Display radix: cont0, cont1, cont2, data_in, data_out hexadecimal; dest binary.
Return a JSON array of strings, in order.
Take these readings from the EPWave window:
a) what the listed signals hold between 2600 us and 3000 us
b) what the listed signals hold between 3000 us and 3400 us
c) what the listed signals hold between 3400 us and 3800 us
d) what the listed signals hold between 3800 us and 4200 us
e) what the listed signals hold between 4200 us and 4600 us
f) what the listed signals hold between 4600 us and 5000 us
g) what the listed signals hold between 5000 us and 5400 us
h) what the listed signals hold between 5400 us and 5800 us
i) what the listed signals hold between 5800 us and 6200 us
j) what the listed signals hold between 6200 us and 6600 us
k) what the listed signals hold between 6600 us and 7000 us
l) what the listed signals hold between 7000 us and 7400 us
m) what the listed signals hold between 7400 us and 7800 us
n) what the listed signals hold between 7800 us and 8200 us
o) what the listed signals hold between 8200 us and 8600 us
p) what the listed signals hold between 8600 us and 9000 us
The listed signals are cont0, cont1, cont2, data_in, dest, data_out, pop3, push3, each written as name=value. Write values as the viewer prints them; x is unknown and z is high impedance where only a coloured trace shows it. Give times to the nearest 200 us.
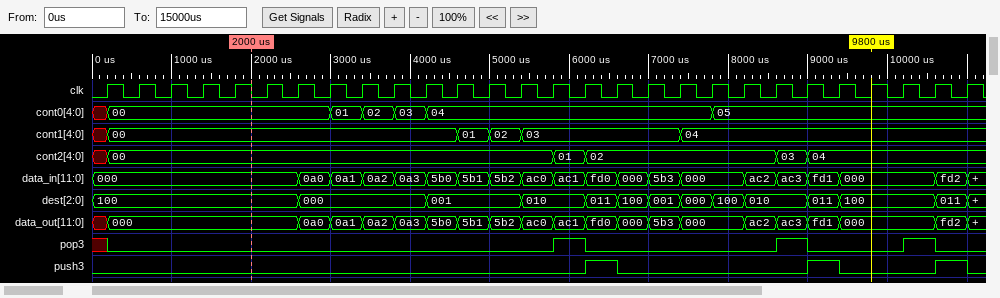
["cont0=00, cont1=00, cont2=00, data_in=0a0, dest=000, data_out=0a0, pop3=0, push3=0", "cont0=01, cont1=00, cont2=00, data_in=0a1, dest=000, data_out=0a1, pop3=0, push3=0", "cont0=02, cont1=00, cont2=00, data_in=0a2, dest=000, data_out=0a2, pop3=0, push3=0", "cont0=03, cont1=00, cont2=00, data_in=0a3, dest=000, data_out=0a3, pop3=0, push3=0", "cont0=04, cont1=00, cont2=00, data_in=5b0, dest=001, data_out=5b0, pop3=0, push3=0", "cont0=04, cont1=01, cont2=00, data_in=5b1, dest=001, data_out=5b1, pop3=0, push3=0", "cont0=04, cont1=02, cont2=00, data_in=5b2, dest=001, data_out=5b2, pop3=0, push3=0", "cont0=04, cont1=03, cont2=00, data_in=ac0, dest=010, data_out=ac0, pop3=0, push3=0", "cont0=04, cont1=03, cont2=01, data_in=ac1, dest=010, data_out=ac1, pop3=1, push3=0", "cont0=04, cont1=03, cont2=02, data_in=fd0, dest=011, data_out=fd0, pop3=0, push3=1", "cont0=04, cont1=03, cont2=02, data_in=000, dest=100, data_out=000, pop3=0, push3=0", "cont0=04, cont1=03, cont2=02, data_in=5b3, dest=001, data_out=5b3, pop3=0, push3=0", "cont0=04, cont1=04, cont2=02, data_in=000, dest=000, data_out=000, pop3=0, push3=0", "cont0=05, cont1=04, cont2=02, data_in=000, dest=100, data_out=000, pop3=0, push3=0", "cont0=05, cont1=04, cont2=02, data_in=ac2, dest=010, data_out=ac2, pop3=0, push3=0", "cont0=05, cont1=04, cont2=03, data_in=ac3, dest=010, data_out=ac3, pop3=1, push3=0"]
